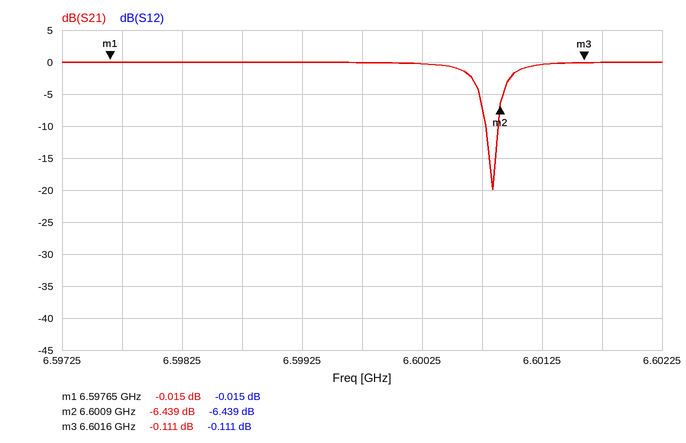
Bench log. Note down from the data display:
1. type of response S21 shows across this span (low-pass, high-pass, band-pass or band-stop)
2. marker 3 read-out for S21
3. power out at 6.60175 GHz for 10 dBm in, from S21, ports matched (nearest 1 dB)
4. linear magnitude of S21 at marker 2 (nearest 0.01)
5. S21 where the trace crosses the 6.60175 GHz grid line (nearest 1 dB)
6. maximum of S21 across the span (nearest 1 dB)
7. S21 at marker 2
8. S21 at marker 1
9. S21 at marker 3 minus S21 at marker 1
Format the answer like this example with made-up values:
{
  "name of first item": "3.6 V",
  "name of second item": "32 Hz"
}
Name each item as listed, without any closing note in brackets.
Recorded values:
{
  "type of response S21 shows across this span": "band-stop",
  "marker 3 read-out for S21": "-0.111 dB",
  "power out at 6.60175 GHz for 10 dBm in, from S21, ports matched": "10 dBm",
  "linear magnitude of S21 at marker 2": "0.48",
  "S21 where the trace crosses the 6.60175 GHz grid line": "0 dB",
  "maximum of S21 across the span": "0 dB",
  "S21 at marker 2": "-6.439 dB",
  "S21 at marker 1": "-0.015 dB",
  "S21 at marker 3 minus S21 at marker 1": "-0.096 dB"
}
